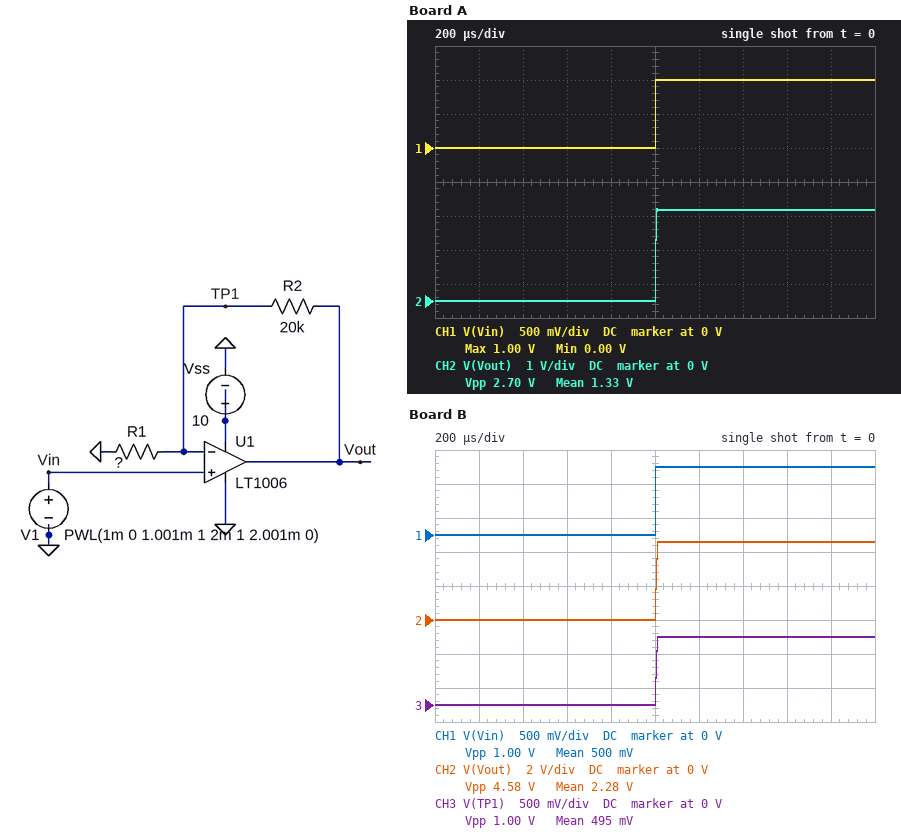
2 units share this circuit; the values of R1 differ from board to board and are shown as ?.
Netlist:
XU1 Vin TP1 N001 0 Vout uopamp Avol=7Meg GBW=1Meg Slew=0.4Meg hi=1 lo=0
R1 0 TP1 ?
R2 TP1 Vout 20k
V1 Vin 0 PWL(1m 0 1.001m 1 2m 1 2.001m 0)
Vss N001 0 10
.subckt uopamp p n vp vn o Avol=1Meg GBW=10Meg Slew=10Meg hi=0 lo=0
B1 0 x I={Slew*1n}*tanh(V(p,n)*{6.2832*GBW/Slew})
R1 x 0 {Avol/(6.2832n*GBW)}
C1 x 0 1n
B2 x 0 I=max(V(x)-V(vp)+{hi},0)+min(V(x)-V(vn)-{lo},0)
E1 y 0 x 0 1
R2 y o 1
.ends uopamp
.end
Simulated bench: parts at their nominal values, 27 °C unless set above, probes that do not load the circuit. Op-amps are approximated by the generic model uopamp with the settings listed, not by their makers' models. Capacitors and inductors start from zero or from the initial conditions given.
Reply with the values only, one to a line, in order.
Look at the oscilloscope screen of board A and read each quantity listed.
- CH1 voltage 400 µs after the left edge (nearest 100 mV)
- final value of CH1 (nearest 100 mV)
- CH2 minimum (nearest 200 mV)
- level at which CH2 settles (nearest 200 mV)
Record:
0 V
1.0 V
0 V
2.6 V
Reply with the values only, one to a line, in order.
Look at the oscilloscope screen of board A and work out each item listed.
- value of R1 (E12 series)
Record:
12 kΩ
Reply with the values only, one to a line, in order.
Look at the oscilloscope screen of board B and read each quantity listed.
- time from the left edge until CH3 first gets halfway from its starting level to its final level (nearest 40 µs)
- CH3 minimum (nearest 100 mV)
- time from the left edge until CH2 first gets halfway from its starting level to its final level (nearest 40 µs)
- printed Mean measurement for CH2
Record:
1.00 ms
0 V
1.00 ms
2.28 V
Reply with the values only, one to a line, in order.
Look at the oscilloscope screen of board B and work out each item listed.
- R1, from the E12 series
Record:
5.6 kΩ
